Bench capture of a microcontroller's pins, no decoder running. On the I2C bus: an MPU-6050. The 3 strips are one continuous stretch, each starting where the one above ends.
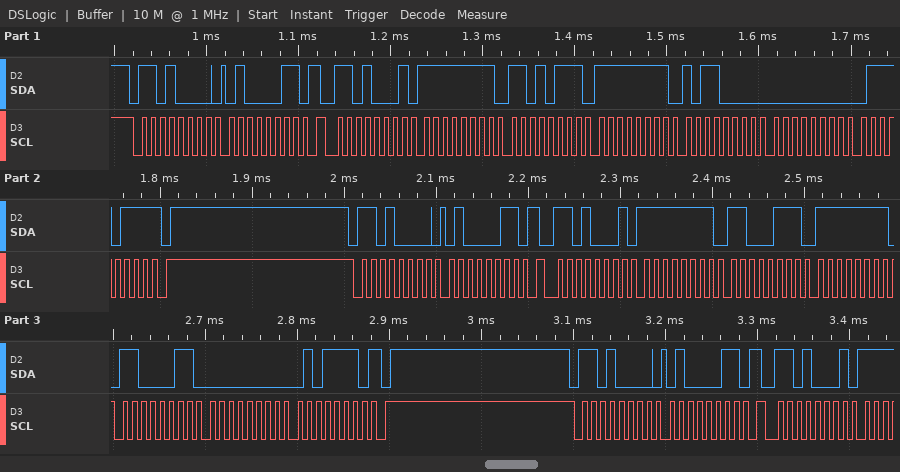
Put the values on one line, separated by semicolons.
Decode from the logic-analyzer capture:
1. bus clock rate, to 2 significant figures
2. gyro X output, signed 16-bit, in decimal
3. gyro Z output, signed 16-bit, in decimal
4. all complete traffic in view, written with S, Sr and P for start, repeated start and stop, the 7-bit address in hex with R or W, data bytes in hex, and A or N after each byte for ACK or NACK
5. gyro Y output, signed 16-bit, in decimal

100 kHz; -41; 119; S 68W A 43 A Sr 68R A FF A D7 A FF A B0 A 00 A 77 N P S 68W A 43 A Sr 68R A FF A C7 A FF A C3 A 00 A 5E N P S 68W A 43 A Sr 68R A; -80
